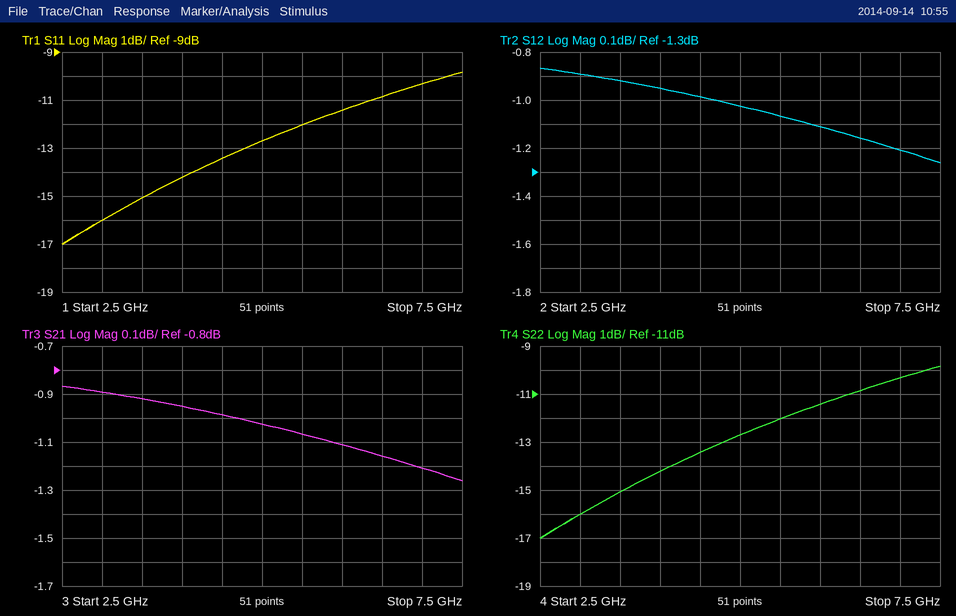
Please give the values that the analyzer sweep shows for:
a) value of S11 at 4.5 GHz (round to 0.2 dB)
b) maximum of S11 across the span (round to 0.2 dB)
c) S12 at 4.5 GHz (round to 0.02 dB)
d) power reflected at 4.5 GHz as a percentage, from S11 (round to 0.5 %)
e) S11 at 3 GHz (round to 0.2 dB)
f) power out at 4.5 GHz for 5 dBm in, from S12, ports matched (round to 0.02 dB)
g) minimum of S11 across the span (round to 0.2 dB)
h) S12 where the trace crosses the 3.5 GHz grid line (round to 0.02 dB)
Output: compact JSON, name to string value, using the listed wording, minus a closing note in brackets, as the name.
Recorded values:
{"value of S11 at 4.5 GHz": "-13.4 dB", "maximum of S11 across the span": "-9.8 dB", "S12 at 4.5 GHz": "-0.98 dB", "power reflected at 4.5 GHz as a percentage, from S11": "4.5 %", "S11 at 3 GHz": "-16.0 dB", "power out at 4.5 GHz for 5 dBm in, from S12, ports matched": "4.02 dBm", "minimum of S11 across the span": "-17.0 dB", "S12 where the trace crosses the 3.5 GHz grid line": "-0.92 dB"}
